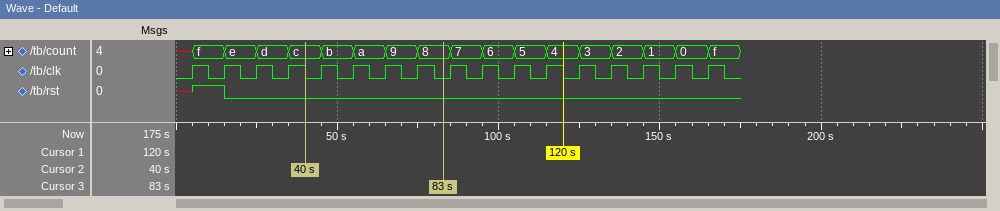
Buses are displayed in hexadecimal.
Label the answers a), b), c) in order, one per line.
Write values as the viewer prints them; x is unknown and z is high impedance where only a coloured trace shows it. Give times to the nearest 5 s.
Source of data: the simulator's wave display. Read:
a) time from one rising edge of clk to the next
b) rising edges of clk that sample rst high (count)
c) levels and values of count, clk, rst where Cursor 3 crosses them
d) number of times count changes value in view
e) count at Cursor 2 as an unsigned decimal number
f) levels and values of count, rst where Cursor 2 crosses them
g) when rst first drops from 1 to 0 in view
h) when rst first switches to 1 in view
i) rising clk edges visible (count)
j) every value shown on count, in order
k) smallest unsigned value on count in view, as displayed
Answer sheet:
a) 10 s
b) 1
c) count=8, clk=0, rst=0
d) 17
e) 12
f) count=c, rst=0
g) 15 s
h) 5 s
i) 17
j) x, f, e, d, c, b, a, 9, 8, 7, 6, 5, 4, 3, 2, 1, 0, f
k) 0
